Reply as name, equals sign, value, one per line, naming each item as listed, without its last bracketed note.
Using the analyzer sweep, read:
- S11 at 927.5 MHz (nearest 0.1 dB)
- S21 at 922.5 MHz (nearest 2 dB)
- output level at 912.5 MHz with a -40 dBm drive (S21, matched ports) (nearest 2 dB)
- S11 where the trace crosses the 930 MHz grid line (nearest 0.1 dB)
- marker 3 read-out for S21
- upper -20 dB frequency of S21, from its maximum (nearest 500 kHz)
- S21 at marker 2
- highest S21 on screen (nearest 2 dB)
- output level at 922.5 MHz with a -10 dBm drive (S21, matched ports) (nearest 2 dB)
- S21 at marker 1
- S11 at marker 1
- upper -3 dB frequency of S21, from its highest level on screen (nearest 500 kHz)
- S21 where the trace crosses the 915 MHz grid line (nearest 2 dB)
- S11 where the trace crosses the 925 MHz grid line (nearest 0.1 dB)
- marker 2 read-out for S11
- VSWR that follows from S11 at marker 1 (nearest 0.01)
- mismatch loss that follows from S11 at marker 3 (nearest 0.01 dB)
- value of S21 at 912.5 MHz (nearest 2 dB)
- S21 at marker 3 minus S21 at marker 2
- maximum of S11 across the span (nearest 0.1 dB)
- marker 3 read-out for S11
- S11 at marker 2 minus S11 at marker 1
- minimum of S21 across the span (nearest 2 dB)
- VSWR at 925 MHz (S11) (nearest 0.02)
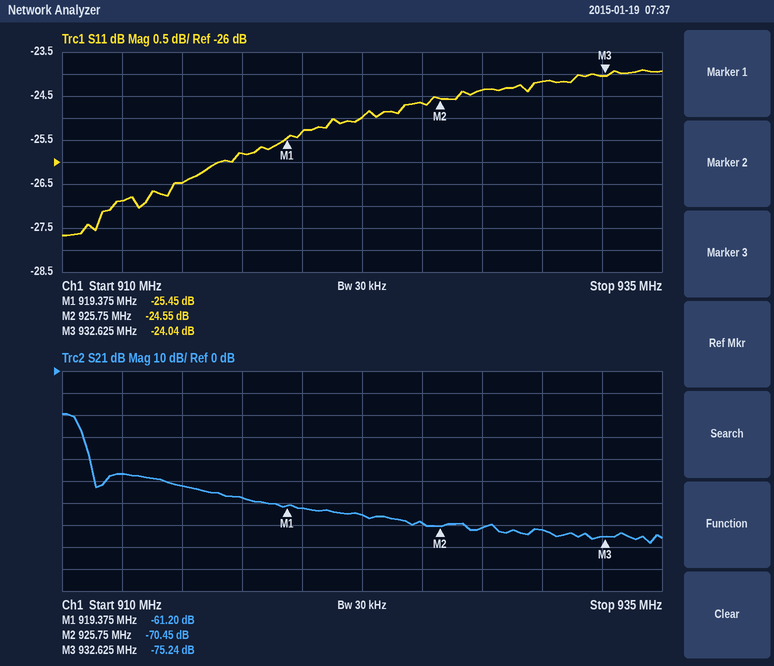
S11 at 927.5 MHz = -24.4 dB
S21 at 922.5 MHz = -66 dB
output level at 912.5 MHz with a -40 dBm drive (S21, matched ports) = -86 dBm
S11 where the trace crosses the 930 MHz grid line = -24.2 dB
marker 3 read-out for S21 = -75.24 dB
upper -20 dB frequency of S21, from its maximum = 911.0 MHz
S21 at marker 2 = -70.45 dB
highest S21 on screen = -20 dB
output level at 922.5 MHz with a -10 dBm drive (S21, matched ports) = -76 dBm
S21 at marker 1 = -61.20 dB
S11 at marker 1 = -25.45 dB
upper -3 dB frequency of S21, from its highest level on screen = 910.5 MHz
S21 where the trace crosses the 915 MHz grid line = -52 dB
S11 where the trace crosses the 925 MHz grid line = -24.7 dB
marker 2 read-out for S11 = -24.55 dB
VSWR that follows from S11 at marker 1 = 1.11
mismatch loss that follows from S11 at marker 3 = 0.02 dB
value of S21 at 912.5 MHz = -46 dB
S21 at marker 3 minus S21 at marker 2 = -4.79 dB
maximum of S11 across the span = -23.9 dB
marker 3 read-out for S11 = -24.04 dB
S11 at marker 2 minus S11 at marker 1 = 0.90 dB
minimum of S21 across the span = -78 dB
VSWR at 925 MHz (S11) = 1.12
